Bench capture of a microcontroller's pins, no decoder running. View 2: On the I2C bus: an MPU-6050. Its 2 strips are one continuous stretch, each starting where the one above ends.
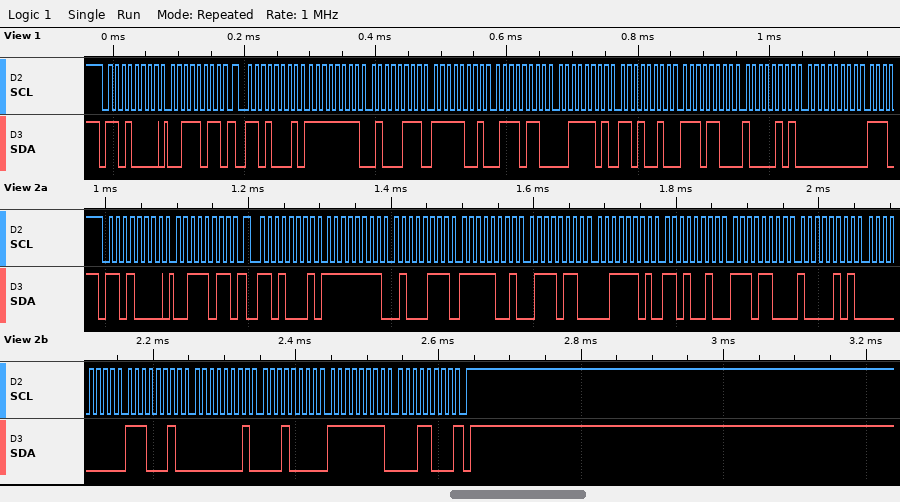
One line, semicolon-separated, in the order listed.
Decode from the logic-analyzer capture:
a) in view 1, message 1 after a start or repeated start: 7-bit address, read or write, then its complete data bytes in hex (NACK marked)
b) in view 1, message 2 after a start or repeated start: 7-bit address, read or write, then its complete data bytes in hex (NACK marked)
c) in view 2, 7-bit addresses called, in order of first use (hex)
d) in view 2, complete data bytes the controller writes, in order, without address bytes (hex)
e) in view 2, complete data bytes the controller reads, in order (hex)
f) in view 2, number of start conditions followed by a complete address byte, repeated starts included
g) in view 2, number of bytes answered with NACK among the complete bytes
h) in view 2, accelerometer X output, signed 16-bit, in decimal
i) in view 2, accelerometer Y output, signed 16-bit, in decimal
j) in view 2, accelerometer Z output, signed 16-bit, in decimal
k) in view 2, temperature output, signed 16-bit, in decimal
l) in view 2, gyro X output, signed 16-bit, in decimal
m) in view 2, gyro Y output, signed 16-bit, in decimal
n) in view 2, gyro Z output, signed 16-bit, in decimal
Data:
0x68 write: 3B; 0x68 read: FF 47 F9 76 3D D2 EC 85 00; 0x68; 3B; FF 47 F9 76 3D D2 EC 85 00 E2 01 10 FF 18; 2; 1; -185; -1674; 15826; -4987; 226; 272; -232
